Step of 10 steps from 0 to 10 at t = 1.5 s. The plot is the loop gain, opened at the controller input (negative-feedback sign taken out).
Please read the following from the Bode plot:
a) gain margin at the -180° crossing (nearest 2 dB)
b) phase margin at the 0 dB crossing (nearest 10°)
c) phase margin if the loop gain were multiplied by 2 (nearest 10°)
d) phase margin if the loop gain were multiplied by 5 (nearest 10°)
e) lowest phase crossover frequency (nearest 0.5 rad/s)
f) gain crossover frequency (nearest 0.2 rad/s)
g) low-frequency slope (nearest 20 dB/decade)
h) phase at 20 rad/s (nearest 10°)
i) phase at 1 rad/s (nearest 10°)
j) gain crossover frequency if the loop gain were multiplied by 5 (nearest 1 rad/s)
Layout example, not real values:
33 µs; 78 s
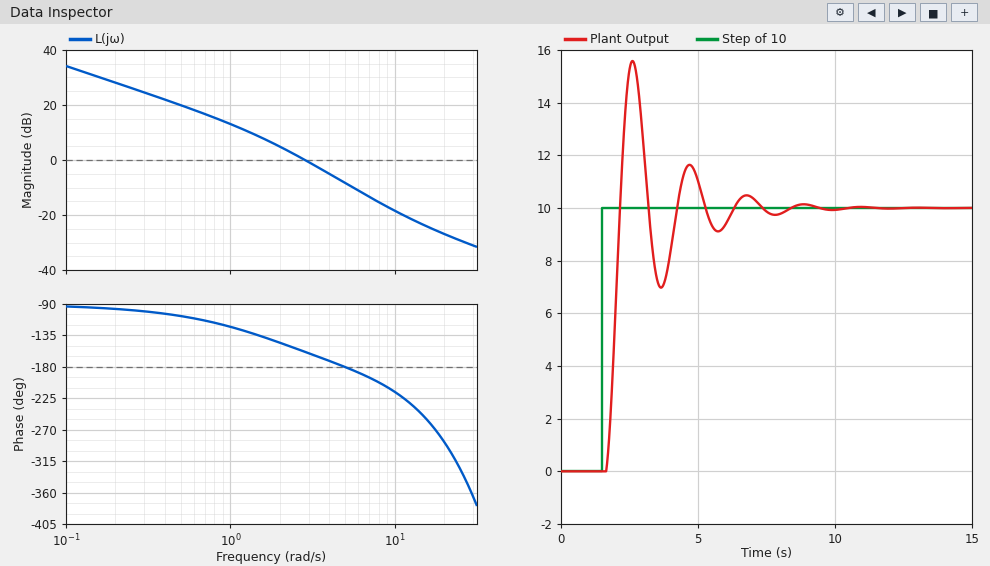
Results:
8 dB; 20°; 10°; -20°; 5.0 rad/s; 2.8 rad/s; -20 dB/decade; -290°; -120°; 7 rad/s
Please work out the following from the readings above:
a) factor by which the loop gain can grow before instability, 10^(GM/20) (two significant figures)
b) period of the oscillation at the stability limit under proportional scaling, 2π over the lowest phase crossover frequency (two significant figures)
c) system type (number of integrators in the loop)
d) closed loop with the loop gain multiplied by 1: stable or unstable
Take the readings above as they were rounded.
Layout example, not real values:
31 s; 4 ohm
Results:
2.5; 1.3 s; 1; stable
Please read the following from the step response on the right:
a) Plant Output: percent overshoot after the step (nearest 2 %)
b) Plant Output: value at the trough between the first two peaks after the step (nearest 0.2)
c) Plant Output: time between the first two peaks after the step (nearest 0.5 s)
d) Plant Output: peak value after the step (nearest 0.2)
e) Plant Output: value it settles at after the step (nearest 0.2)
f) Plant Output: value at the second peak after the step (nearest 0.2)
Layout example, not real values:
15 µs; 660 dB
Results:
56 %; 7.0; 2.0 s; 15.6; 10.0; 11.6
